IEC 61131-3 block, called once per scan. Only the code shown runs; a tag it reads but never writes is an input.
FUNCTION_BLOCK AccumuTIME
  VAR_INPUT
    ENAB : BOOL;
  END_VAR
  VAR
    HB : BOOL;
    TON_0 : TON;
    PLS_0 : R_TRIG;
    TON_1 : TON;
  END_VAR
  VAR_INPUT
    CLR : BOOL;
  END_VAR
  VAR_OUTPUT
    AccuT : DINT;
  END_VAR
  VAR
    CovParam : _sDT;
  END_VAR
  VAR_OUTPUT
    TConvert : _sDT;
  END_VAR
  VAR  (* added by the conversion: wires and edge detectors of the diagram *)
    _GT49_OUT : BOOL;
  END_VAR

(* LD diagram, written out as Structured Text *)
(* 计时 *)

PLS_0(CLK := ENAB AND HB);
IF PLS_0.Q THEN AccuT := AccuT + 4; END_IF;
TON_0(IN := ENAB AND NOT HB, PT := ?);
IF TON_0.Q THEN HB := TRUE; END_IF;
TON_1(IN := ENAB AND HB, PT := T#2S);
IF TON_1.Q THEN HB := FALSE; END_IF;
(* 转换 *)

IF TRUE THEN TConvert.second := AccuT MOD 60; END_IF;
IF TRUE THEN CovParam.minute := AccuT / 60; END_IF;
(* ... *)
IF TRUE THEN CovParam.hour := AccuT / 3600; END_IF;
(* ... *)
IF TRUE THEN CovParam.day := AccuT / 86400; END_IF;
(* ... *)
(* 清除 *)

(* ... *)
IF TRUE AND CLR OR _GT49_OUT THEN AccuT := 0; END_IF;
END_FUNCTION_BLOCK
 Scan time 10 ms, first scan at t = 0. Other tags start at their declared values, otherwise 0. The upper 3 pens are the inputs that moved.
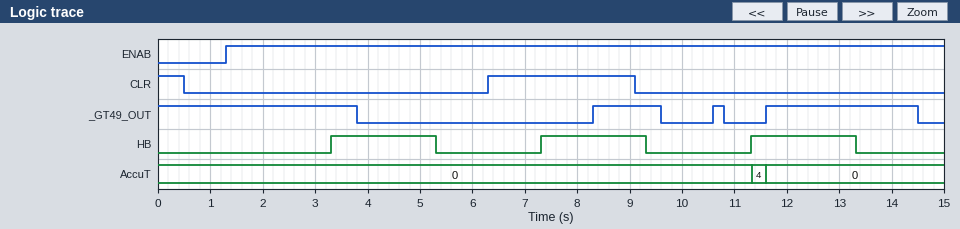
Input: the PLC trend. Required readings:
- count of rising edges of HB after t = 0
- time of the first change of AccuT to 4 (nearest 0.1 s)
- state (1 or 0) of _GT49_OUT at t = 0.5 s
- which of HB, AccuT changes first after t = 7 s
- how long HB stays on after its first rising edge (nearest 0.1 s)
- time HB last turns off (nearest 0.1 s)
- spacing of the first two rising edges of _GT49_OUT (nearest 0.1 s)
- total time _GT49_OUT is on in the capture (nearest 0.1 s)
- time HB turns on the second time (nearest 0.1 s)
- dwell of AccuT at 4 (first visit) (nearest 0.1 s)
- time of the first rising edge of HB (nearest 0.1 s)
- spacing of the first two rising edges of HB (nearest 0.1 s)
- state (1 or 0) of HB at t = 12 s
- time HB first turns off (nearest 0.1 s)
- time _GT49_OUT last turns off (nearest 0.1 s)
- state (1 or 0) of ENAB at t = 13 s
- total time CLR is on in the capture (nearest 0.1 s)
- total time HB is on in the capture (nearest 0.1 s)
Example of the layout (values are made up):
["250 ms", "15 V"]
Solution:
["3", "11.3 s", "1", "HB", "2.0 s", "13.3 s", "2.3 s", "8.2 s", "7.3 s", "0.3 s", "3.3 s", "4.0 s", "1", "5.3 s", "14.5 s", "1", "3.3 s", "6.0 s"]
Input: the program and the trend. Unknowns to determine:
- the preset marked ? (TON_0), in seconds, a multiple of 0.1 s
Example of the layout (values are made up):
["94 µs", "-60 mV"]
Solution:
["2.0 s"]
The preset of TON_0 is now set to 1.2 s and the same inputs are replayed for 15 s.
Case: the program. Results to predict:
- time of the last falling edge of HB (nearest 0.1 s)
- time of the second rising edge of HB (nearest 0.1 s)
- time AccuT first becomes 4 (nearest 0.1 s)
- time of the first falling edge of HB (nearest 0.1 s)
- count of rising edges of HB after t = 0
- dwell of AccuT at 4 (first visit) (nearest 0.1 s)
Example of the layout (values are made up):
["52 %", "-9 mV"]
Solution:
["14.1 s", "5.7 s", "5.7 s", "4.5 s", "4", "0.6 s"]
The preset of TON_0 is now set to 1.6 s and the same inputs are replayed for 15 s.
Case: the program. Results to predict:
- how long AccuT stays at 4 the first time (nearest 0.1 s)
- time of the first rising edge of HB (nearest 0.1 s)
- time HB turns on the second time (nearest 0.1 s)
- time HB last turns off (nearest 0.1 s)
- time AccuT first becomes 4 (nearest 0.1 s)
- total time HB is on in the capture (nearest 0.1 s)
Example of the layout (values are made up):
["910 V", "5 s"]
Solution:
["0.5 s", "2.9 s", "6.5 s", "12.1 s", "10.1 s", "7.3 s"]
